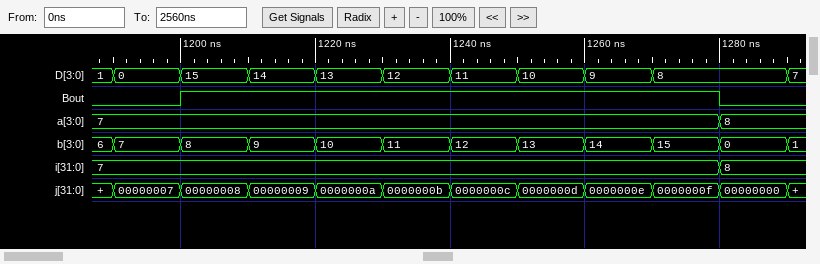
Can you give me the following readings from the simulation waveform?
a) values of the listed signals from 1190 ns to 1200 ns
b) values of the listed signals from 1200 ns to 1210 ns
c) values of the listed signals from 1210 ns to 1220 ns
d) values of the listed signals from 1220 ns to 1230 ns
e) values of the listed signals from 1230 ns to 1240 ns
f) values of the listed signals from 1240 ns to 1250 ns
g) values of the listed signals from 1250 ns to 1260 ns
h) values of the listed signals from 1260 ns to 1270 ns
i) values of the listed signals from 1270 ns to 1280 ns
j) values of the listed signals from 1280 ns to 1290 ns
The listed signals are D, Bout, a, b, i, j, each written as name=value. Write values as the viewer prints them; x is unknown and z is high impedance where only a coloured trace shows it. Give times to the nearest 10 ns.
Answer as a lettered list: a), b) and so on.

a) D=0, Bout=0, a=7, b=7, i=7, j=00000007
b) D=15, Bout=1, a=7, b=8, i=7, j=00000008
c) D=14, Bout=1, a=7, b=9, i=7, j=00000009
d) D=13, Bout=1, a=7, b=10, i=7, j=0000000a
e) D=12, Bout=1, a=7, b=11, i=7, j=0000000b
f) D=11, Bout=1, a=7, b=12, i=7, j=0000000c
g) D=10, Bout=1, a=7, b=13, i=7, j=0000000d
h) D=9, Bout=1, a=7, b=14, i=7, j=0000000e
i) D=8, Bout=1, a=7, b=15, i=7, j=0000000f
j) D=8, Bout=0, a=8, b=0, i=8, j=00000000
